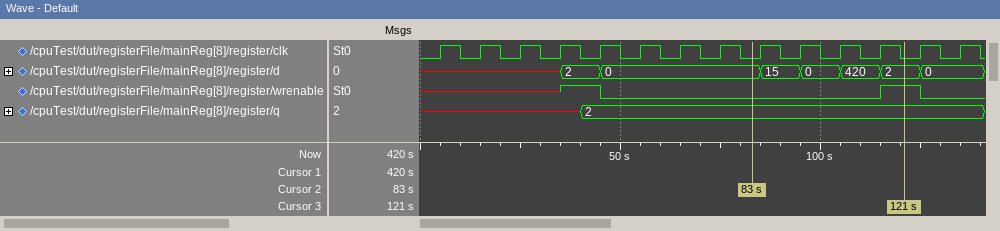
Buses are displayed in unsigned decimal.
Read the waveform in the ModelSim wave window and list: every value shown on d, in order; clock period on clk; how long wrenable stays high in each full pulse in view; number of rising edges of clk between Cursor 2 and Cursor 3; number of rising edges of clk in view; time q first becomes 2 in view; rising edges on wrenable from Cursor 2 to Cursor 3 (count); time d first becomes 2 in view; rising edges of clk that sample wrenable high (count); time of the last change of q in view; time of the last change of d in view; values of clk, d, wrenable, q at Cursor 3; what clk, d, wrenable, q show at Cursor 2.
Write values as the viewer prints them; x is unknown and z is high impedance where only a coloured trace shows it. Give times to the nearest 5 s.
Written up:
x, 2, 0, 15, 0, 420, 2, 0
10 s
10 s
4
14
40 s
1
35 s
2
40 s
125 s
clk=0, d=2, wrenable=1, q=2
clk=0, d=0, wrenable=0, q=2
